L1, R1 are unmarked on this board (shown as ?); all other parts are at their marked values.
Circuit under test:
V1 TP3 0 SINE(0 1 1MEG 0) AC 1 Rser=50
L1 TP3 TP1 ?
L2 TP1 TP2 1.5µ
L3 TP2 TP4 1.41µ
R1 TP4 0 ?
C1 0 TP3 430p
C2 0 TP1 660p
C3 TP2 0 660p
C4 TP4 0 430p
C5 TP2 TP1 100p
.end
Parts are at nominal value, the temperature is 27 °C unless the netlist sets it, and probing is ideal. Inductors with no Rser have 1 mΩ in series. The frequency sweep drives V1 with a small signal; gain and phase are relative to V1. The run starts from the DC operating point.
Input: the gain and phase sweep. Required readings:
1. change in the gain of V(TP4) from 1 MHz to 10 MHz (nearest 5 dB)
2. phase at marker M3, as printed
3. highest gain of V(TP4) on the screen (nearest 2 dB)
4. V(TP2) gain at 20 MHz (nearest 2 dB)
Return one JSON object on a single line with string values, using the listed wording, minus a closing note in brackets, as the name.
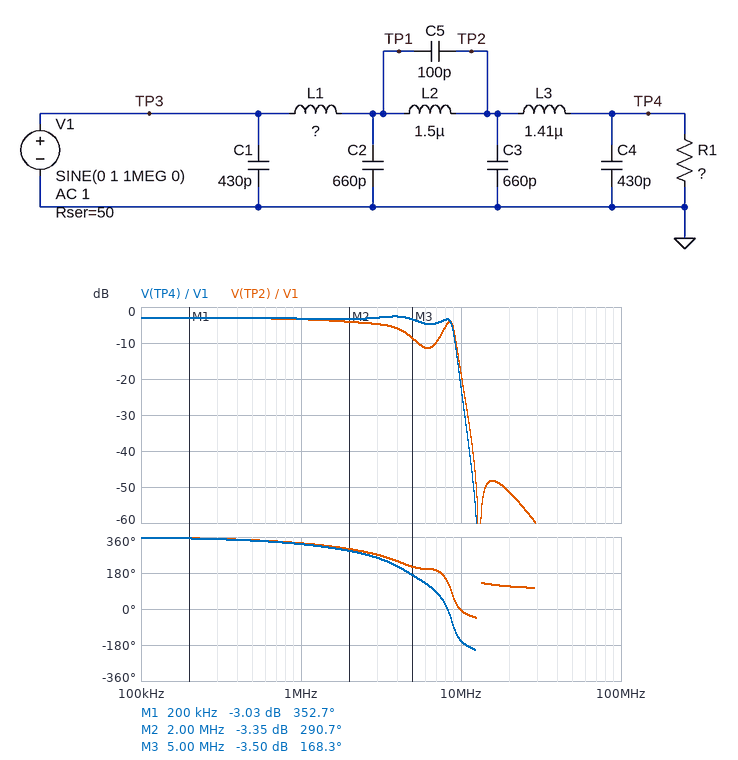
{"change in the gain of V(TP4) from 1 MHz to 10 MHz": "-20 dB", "phase at marker M3, as printed": "168.3 deg", "highest gain of V(TP4) on the screen": "-2 dB", "V(TP2) gain at 20 MHz": "-52 dB"}
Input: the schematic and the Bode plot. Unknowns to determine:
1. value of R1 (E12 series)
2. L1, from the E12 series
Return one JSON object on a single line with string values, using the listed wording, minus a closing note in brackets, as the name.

{"value of R1": "120 Ω", "L1, from the E12 series": "1.2 µH"}
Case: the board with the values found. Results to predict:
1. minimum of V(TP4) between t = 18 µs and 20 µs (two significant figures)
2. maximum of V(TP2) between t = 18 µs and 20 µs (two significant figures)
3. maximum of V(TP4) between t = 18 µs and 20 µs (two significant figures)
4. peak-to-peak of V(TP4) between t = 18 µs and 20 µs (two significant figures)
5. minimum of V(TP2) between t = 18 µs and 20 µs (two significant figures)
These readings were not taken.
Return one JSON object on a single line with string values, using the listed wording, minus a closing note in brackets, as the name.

{"minimum of V(TP4) between t = 18 µs and 20 µs": "-690 mV", "maximum of V(TP2) between t = 18 µs and 20 µs": "680 mV", "maximum of V(TP4) between t = 18 µs and 20 µs": "690 mV", "peak-to-peak of V(TP4) between t = 18 µs and 20 µs": "1.4 V", "minimum of V(TP2) between t = 18 µs and 20 µs": "-680 mV"}
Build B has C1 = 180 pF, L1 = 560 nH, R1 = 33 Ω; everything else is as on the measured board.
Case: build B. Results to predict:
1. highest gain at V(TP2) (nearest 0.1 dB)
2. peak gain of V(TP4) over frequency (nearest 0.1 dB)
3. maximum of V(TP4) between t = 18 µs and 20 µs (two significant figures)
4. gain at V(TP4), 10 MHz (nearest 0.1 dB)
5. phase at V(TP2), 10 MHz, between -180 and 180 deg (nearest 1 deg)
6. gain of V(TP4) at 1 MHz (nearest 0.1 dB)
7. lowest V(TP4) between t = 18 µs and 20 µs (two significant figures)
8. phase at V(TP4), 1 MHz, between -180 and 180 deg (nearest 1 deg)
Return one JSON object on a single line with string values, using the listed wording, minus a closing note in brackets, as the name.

{"highest gain at V(TP2)": "-3.0 dB", "peak gain of V(TP4) over frequency": "-7.9 dB", "maximum of V(TP4) between t = 18 µs and 20 µs": "400 mV", "gain at V(TP4), 10 MHz": "-29.2 dB", "phase at V(TP2), 10 MHz, between -180 and 180 deg": "88 deg", "gain of V(TP4) at 1 MHz": "-8.0 dB", "lowest V(TP4) between t = 18 µs and 20 µs": "-400 mV", "phase at V(TP4), 1 MHz, between -180 and 180 deg": "-29 deg"}
